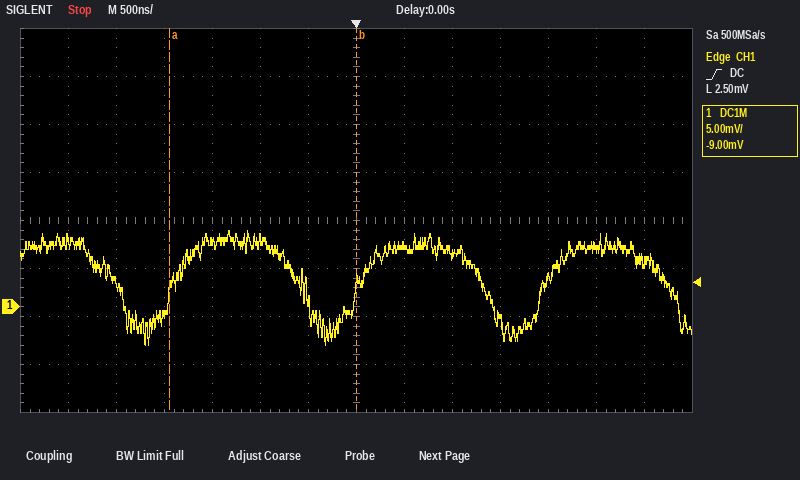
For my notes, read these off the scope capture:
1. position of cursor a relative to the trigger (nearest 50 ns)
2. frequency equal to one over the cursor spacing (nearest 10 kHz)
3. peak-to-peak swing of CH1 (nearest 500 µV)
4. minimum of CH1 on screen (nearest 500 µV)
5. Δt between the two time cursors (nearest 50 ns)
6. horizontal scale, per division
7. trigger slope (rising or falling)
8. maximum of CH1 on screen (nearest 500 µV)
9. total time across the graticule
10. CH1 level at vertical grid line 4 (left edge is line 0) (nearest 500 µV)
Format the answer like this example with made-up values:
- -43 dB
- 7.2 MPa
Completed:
- -1.95 µs
- 510 kHz
- 12.0 mV
- -4.0 mV
- 1.95 µs
- 500 ns
- rising
- 8.0 mV
- 7 µs
- 7.0 mV
